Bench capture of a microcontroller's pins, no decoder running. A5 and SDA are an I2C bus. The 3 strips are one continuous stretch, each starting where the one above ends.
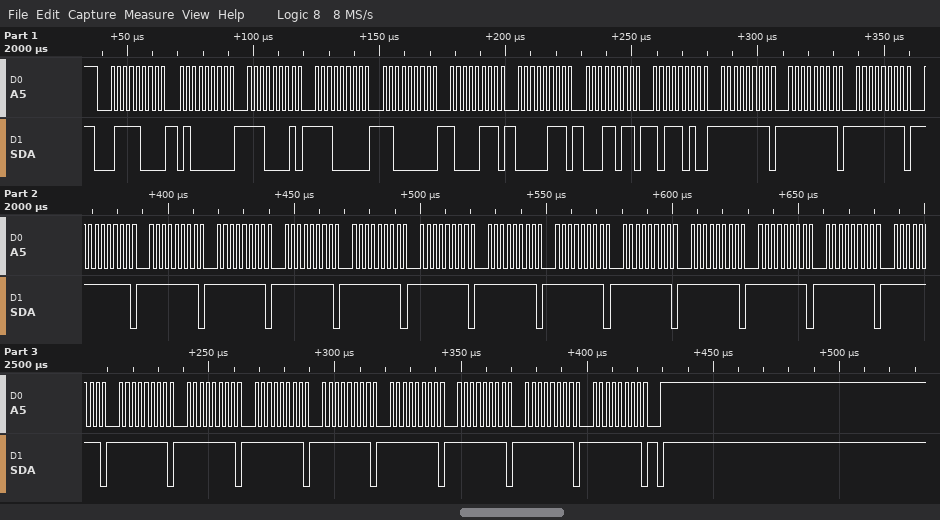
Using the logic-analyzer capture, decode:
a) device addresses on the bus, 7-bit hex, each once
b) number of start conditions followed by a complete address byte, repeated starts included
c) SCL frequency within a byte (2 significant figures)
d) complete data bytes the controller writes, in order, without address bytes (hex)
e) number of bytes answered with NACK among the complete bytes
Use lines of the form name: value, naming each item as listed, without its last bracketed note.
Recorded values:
device addresses on the bus, 7-bit hex, each once: 0x3C
number of start conditions followed by a complete address byte, repeated starts included: 1
SCL frequency within a byte: 400 kHz
complete data bytes the controller writes, in order, without address bytes: 40 E1 E0 C0 87 07 1B BA FF FF FF FF FF FF FF FF FF FF FF FF FF FF FF FF FF FF FF FF FF FF FF FF
number of bytes answered with NACK among the complete bytes: 0
